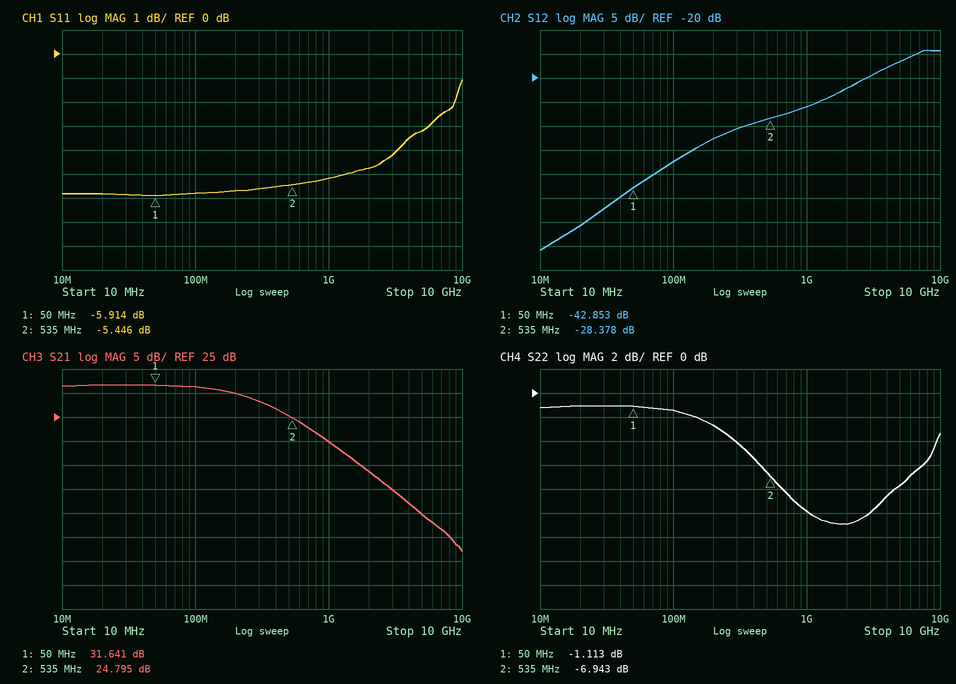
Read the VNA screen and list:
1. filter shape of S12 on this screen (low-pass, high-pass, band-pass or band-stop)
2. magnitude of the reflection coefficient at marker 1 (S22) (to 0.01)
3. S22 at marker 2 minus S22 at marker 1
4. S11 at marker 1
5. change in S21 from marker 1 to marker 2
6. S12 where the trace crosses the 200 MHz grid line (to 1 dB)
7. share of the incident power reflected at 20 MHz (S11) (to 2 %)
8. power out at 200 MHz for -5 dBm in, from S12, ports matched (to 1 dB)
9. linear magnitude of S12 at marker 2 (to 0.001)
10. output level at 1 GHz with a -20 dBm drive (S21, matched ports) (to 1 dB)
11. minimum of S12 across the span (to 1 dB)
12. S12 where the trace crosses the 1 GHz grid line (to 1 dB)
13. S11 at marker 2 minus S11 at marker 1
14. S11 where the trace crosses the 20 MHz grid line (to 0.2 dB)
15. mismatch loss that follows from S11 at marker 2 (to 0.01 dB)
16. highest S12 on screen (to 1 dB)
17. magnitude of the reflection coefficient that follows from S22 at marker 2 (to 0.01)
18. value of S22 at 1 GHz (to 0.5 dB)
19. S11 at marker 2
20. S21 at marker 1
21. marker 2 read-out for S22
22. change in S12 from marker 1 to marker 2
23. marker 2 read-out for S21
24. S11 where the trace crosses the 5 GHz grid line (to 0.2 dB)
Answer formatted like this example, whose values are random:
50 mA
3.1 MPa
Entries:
high-pass
0.88
-5.830 dB
-5.914 dB
-6.846 dB
-33 dB
26 %
-38 dBm
0.038
0 dBm
-56 dB
-26 dB
0.468 dB
-5.8 dB
1.46 dB
-14 dB
0.45
-10.0 dB
-5.446 dB
31.641 dB
-6.943 dB
14.475 dB
24.795 dB
-3.2 dB
